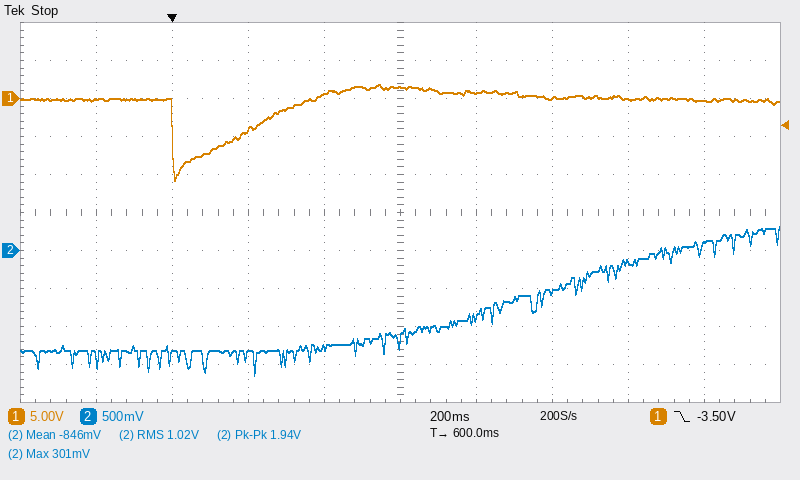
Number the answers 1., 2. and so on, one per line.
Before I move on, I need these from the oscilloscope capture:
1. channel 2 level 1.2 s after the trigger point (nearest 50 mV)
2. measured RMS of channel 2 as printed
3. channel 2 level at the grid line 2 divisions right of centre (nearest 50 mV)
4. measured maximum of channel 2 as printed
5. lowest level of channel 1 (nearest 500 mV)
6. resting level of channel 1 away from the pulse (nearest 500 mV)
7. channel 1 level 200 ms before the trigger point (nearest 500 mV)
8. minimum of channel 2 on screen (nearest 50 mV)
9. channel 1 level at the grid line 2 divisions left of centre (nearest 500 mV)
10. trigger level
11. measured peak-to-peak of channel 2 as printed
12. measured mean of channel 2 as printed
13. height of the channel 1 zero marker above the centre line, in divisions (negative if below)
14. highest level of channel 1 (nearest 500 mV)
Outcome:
1. -150 mV
2. 1.02 V
3. -550 mV
4. 301 mV
5. -11.0 V
6. 0.0 V
7. 0.0 V
8. -1.65 V
9. -4.0 V
10. -3.50 V
11. 1.94 V
12. -846 mV
13. +3.0 div
14. 2.0 V
